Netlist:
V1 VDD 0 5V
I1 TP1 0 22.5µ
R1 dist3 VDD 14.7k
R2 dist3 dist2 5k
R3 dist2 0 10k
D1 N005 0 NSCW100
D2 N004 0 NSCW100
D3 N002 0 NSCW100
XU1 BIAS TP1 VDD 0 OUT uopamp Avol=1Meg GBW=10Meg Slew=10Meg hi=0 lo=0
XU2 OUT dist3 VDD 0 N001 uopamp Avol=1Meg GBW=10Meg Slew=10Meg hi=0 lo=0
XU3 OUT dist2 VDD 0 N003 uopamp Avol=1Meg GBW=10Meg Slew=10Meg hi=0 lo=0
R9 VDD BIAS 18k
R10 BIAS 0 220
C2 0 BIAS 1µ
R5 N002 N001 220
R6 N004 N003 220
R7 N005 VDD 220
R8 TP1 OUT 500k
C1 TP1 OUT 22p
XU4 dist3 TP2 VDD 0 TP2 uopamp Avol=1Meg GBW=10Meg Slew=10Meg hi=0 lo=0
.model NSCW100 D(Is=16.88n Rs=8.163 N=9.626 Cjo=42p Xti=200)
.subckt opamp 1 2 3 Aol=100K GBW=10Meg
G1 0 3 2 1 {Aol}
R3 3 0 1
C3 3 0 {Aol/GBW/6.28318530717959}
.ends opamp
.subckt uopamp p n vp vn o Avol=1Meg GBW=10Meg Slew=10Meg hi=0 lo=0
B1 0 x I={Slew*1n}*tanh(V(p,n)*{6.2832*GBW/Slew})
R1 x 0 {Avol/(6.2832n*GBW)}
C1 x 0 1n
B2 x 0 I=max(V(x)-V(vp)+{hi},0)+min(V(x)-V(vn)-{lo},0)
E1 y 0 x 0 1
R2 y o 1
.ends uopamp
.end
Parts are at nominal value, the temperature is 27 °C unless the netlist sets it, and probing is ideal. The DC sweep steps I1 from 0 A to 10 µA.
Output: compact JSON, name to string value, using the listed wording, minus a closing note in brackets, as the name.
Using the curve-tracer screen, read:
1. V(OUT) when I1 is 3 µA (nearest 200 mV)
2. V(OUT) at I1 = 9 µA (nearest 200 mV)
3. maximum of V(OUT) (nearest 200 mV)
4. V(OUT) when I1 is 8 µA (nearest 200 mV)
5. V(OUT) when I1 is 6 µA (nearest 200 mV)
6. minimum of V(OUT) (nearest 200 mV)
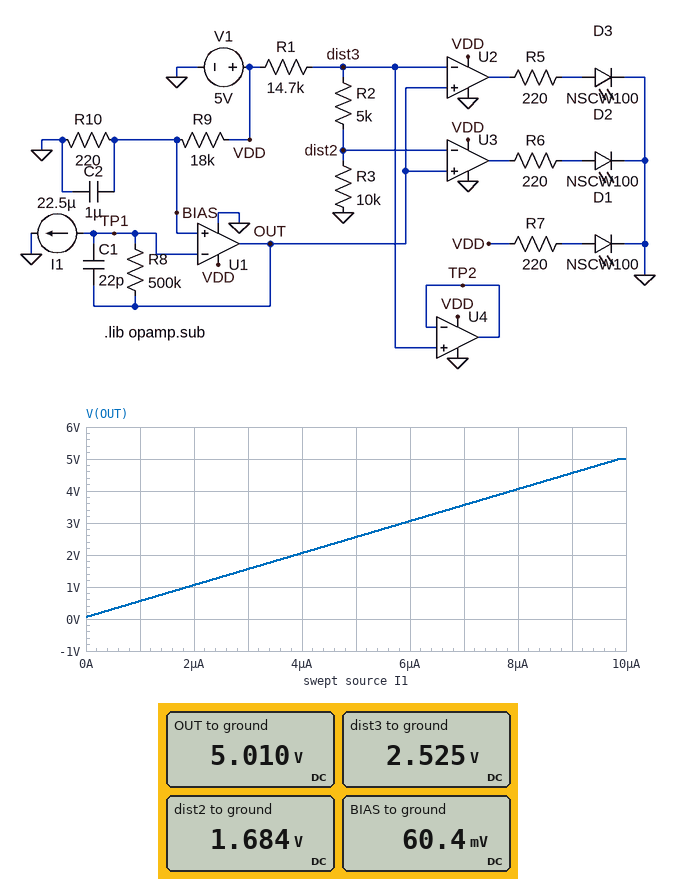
{"V(OUT) when I1 is 3 µA": "1.6 V", "V(OUT) at I1 = 9 µA": "4.6 V", "maximum of V(OUT)": "5.0 V", "V(OUT) when I1 is 8 µA": "4.0 V", "V(OUT) when I1 is 6 µA": "3.0 V", "minimum of V(OUT)": "0 V"}
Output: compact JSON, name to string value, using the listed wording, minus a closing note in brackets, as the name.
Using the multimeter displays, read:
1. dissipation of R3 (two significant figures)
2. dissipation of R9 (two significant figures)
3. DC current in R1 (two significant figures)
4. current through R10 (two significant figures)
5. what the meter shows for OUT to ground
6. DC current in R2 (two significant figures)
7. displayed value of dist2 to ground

{"dissipation of R3": "280 µW", "dissipation of R9": "1.4 mW", "DC current in R1": "170 µA", "current through R10": "270 µA", "what the meter shows for OUT to ground": "5.010 V", "DC current in R2": "170 µA", "displayed value of dist2 to ground": "1.684 V"}
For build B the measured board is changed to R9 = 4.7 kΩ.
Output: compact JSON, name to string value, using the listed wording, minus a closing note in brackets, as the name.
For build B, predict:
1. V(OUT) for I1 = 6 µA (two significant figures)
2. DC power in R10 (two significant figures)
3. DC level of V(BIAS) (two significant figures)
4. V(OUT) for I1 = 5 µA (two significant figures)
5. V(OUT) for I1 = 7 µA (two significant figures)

{"V(OUT) for I1 = 6 µA": "3.2 V", "DC power in R10": "230 µW", "DC level of V(BIAS)": "220 mV", "V(OUT) for I1 = 5 µA": "2.7 V", "V(OUT) for I1 = 7 µA": "3.7 V"}
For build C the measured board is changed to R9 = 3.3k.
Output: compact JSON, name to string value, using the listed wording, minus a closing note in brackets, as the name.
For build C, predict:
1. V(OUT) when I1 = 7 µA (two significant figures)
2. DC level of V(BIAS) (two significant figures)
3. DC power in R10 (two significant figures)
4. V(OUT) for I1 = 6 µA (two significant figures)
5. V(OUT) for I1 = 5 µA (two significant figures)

{"V(OUT) when I1 = 7 µA": "3.8 V", "DC level of V(BIAS)": "310 mV", "DC power in R10": "440 µW", "V(OUT) for I1 = 6 µA": "3.3 V", "V(OUT) for I1 = 5 µA": "2.8 V"}
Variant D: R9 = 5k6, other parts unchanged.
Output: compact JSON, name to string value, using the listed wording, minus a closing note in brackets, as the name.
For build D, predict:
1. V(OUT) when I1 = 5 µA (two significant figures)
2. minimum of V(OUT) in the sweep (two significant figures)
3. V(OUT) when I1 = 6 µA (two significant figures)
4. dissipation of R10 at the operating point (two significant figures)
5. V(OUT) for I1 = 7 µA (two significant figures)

{"V(OUT) when I1 = 5 µA": "2.7 V", "minimum of V(OUT) in the sweep": "190 mV", "V(OUT) when I1 = 6 µA": "3.2 V", "dissipation of R10 at the operating point": "160 µW", "V(OUT) for I1 = 7 µA": "3.7 V"}
